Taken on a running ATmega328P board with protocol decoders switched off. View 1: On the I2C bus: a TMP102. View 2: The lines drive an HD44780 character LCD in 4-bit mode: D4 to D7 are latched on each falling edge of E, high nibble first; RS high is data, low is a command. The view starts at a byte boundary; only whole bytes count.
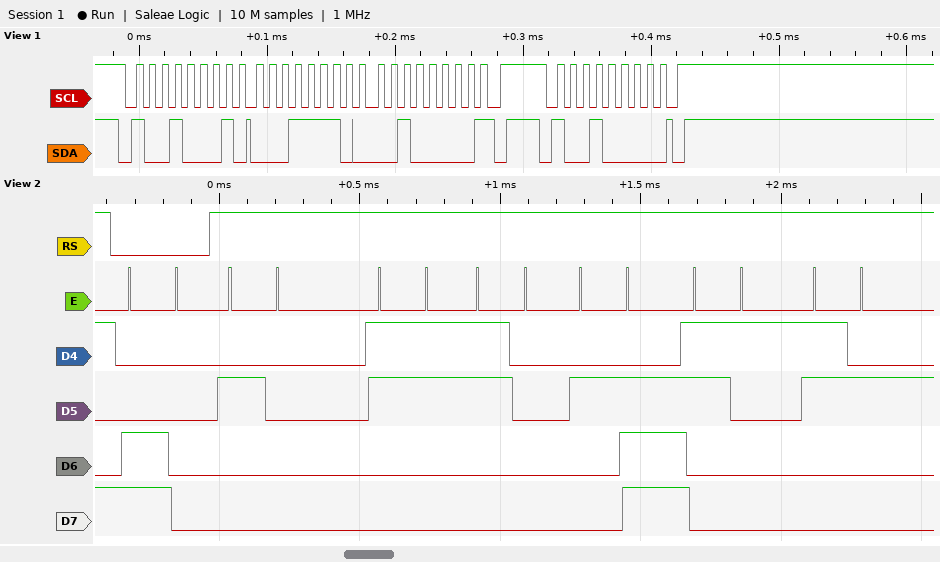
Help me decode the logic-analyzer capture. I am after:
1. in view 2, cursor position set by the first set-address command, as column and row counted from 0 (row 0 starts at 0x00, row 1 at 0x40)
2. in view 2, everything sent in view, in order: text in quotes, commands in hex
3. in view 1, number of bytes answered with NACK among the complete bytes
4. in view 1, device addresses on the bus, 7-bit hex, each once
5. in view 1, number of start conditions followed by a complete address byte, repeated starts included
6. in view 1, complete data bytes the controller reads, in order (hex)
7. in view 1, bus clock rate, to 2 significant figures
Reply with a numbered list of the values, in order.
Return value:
1. column 0, row 1
2. 0xC0 " 30.12"
3. 1
4. 0x48
5. 2
6. 1E 20
7. 100 kHz
